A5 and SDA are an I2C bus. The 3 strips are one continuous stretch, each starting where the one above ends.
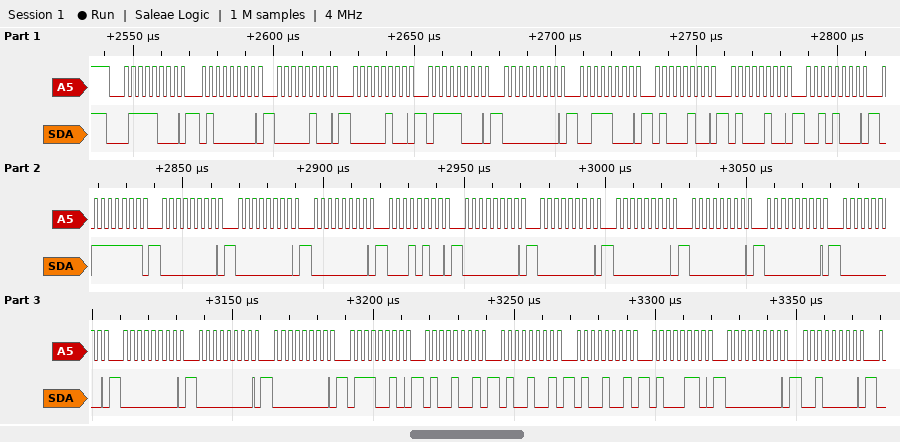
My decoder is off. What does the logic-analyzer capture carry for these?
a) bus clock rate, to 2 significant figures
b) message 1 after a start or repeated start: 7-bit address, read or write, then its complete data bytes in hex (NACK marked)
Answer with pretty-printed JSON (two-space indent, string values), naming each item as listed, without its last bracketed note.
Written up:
{
  "bus clock rate, to 2 significant figures": "400 kHz",
  "message 1 after a start or repeated start: 7-bit address, read or write, then its complete data bytes in hex": "0x3C write: 40 04 04 78 00 38 44 44 28 7F 00 00 00 14 00 00 00 00 00 00 00 00 00 72 49 49 49 46 00 20"
}
